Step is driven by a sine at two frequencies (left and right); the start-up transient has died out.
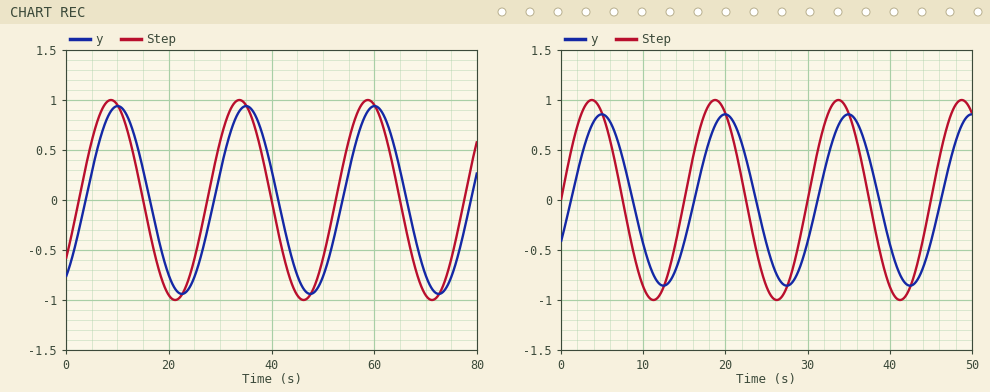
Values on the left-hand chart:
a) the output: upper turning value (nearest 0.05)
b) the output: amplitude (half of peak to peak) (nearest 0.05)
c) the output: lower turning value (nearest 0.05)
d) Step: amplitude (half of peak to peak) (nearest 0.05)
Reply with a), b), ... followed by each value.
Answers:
a) 0.95
b) 0.95
c) -0.95
d) 1.00
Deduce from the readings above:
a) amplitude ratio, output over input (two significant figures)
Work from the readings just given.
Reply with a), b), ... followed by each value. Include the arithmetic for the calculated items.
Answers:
a) 0.95 / 1 = 0.95
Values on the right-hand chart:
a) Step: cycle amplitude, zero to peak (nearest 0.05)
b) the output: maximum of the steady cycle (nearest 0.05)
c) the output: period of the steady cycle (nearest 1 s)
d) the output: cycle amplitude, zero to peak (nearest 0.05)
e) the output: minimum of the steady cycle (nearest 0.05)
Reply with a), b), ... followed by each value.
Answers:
a) 1.00
b) 0.85
c) 15 s
d) 0.85
e) -0.85
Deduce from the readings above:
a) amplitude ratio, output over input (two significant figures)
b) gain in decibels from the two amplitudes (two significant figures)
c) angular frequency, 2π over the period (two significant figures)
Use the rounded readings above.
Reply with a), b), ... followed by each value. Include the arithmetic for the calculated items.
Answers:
a) 0.85 / 1 = 0.85
b) 20 log10(0.85 / 1) = -1.4 dB
c) 2π / 15 = 0.42 rad/s
